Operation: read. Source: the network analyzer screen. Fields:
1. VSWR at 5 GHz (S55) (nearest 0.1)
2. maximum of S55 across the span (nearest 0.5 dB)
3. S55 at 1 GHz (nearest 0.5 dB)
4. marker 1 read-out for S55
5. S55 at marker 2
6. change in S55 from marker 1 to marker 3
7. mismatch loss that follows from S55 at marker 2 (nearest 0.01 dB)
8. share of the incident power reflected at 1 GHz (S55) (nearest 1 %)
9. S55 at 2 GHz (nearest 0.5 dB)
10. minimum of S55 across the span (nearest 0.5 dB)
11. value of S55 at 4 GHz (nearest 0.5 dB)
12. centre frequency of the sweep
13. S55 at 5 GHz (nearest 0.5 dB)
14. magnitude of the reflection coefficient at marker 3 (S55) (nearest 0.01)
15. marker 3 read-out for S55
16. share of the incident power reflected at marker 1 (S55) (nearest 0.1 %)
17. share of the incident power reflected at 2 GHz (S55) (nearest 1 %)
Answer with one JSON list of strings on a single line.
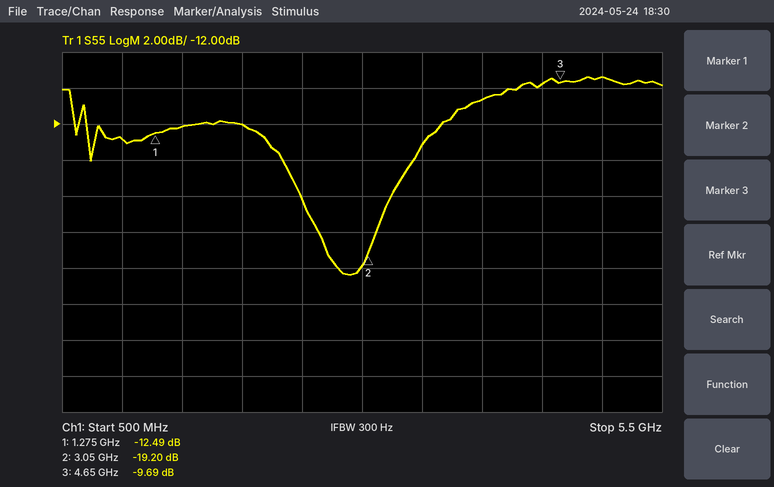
["2.0", "-9.5 dB", "-13.0 dB", "-12.49 dB", "-19.20 dB", "2.80 dB", "0.05 dB", "5 %", "-12.0 dB", "-20.5 dB", "-10.5 dB", "3 GHz", "-9.5 dB", "0.33", "-9.69 dB", "5.6 %", "6 %"]
